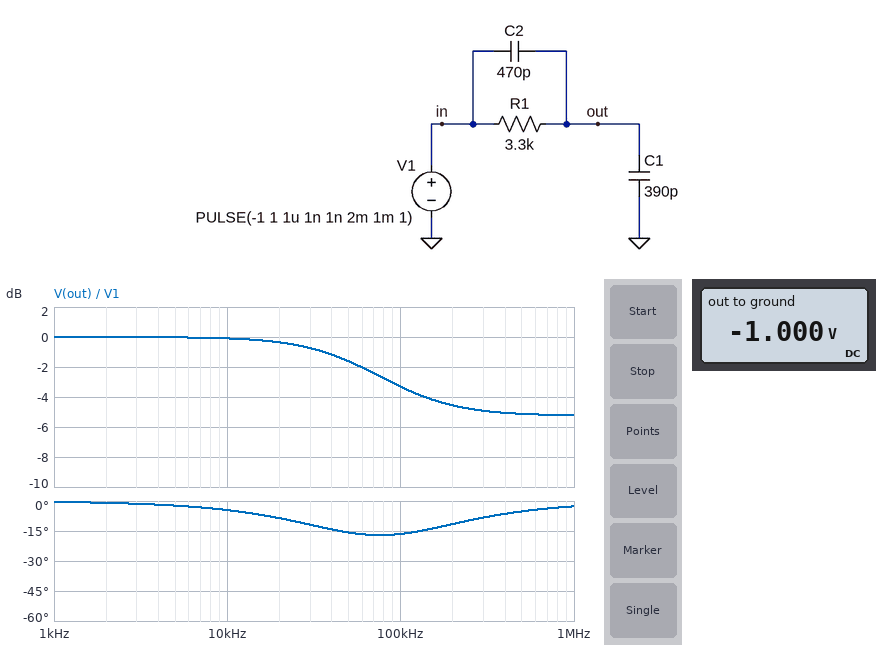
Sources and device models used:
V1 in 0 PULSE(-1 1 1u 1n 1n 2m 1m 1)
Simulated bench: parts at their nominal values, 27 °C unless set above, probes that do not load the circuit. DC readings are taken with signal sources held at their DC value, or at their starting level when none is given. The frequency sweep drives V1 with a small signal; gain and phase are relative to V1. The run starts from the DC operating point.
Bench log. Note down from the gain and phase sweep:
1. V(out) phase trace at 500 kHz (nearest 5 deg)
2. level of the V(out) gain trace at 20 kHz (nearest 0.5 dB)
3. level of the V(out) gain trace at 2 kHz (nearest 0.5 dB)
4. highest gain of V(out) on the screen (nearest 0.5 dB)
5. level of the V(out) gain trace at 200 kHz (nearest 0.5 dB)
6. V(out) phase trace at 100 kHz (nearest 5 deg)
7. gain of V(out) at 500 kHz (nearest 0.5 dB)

-5 deg
-0.5 dB
0 dB
0 dB
-4.5 dB
-15 deg
-5.0 dB
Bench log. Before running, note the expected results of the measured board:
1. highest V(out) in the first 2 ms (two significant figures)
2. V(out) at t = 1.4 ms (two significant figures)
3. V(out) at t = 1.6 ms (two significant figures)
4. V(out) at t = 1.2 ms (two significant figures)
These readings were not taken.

1.0 V
-1.0 V
-1.0 V
-1.0 V
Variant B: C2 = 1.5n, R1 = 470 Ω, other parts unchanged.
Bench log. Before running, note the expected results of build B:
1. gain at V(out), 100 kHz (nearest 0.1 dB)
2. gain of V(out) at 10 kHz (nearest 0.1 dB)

-0.4 dB
0 dB
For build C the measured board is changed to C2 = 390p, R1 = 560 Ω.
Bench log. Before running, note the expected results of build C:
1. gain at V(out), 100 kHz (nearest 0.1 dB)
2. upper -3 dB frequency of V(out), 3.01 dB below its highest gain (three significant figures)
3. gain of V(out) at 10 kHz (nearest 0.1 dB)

-0.2 dB
515 kHz
0 dB
